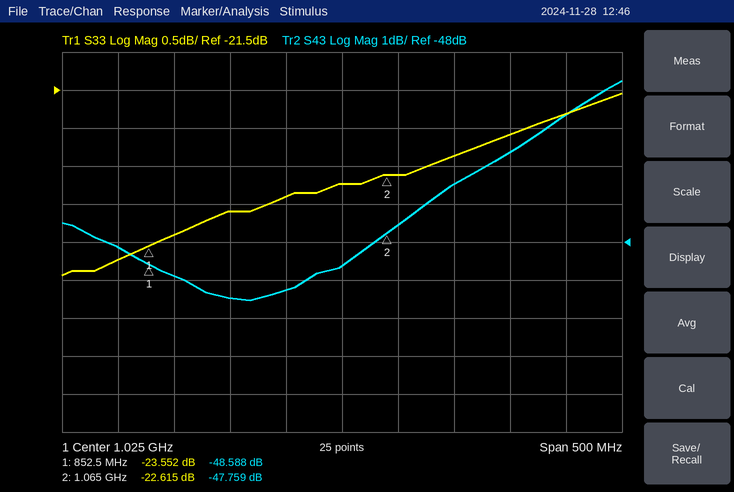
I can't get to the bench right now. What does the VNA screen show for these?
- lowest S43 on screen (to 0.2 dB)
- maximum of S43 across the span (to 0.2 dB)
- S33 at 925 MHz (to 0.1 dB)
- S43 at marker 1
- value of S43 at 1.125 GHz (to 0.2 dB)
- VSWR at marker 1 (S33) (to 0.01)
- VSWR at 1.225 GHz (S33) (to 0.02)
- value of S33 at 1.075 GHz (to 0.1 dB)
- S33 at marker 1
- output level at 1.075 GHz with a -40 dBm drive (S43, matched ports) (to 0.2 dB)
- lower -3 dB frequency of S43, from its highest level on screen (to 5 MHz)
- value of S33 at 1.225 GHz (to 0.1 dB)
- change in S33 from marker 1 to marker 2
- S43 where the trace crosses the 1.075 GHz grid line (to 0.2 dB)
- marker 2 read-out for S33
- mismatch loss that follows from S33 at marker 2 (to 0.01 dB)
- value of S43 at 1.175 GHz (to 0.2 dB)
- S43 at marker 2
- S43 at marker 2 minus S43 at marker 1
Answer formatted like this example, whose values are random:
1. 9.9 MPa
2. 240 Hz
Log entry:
1. -49.6 dB
2. -43.8 dB
3. -23.1 dB
4. -48.588 dB
5. -46.4 dB
6. 1.14
7. 1.18
8. -22.6 dB
9. -23.552 dB
10. -87.6 dBm
11. 1.110 GHz
12. -21.8 dB
13. 0.937 dB
14. -47.6 dB
15. -22.615 dB
16. 0.02 dB
17. -45.6 dB
18. -47.759 dB
19. 0.829 dB
